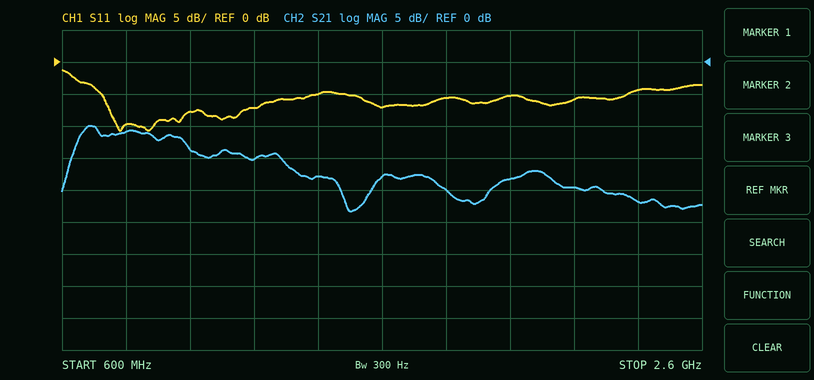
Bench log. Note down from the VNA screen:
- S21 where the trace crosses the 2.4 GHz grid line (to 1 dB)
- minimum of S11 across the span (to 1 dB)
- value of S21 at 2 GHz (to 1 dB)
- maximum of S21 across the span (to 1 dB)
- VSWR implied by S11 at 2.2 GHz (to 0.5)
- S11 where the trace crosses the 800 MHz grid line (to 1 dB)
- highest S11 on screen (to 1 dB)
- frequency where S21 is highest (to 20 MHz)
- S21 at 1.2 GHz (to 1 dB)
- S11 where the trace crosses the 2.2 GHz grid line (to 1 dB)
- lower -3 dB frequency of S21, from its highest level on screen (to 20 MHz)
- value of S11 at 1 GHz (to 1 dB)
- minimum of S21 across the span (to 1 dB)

-22 dB
-11 dB
-18 dB
-10 dB
3.0
-10 dB
-1 dB
680 MHz
-15 dB
-6 dB
640 MHz
-8 dB
-23 dB
